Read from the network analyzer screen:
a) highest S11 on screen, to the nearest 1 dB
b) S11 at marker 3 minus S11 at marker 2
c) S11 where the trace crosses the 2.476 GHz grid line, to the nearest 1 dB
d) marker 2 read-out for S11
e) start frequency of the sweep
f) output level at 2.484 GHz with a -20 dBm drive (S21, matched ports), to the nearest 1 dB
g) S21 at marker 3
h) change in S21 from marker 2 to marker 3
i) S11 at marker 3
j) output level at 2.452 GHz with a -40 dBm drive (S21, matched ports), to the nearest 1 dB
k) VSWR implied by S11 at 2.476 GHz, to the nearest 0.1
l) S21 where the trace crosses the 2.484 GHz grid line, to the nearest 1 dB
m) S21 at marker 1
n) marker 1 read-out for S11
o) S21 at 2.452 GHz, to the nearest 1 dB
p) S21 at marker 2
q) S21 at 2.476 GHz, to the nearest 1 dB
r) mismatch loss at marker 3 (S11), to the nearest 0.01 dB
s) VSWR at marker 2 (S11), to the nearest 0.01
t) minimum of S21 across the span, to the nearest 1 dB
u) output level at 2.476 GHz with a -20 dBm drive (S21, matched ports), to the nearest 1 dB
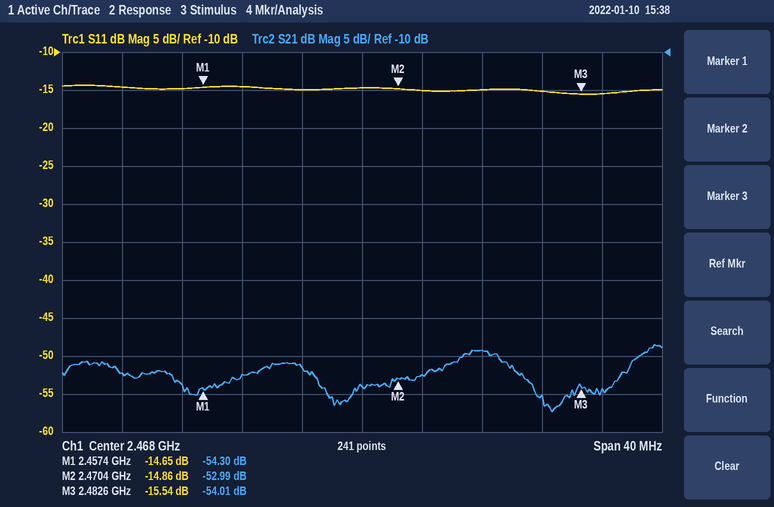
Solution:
-14 dB
-0.68 dB
-15 dB
-14.86 dB
2.448 GHz
-74 dBm
-54.01 dB
-1.02 dB
-15.54 dB
-92 dBm
1.4
-54 dB
-54.30 dB
-14.65 dB
-52 dB
-52.99 dB
-49 dB
0.12 dB
1.44
-57 dB
-69 dBm
